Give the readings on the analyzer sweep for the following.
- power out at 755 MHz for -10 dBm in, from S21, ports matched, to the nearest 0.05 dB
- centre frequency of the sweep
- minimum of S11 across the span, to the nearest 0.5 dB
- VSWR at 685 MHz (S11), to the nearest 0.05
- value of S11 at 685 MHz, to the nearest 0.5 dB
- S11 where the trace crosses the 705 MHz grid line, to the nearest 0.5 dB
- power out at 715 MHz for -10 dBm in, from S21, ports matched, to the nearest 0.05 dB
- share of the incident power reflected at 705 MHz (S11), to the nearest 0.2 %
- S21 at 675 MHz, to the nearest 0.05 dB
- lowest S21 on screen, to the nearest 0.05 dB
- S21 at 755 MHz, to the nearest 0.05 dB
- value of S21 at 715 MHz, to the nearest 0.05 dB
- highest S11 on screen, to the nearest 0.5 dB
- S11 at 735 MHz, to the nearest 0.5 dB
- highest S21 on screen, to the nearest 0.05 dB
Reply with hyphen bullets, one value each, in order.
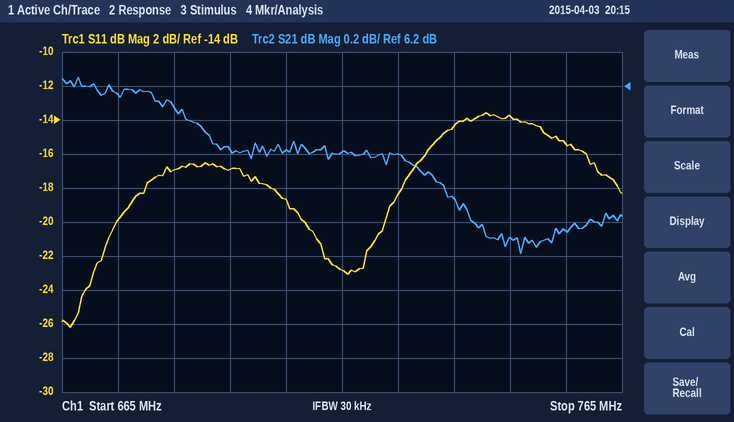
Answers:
- -4.65 dBm
- 715 MHz
- -26.0 dB
- 1.35
- -17.0 dB
- -18.5 dB
- -4.20 dBm
- 1.4 %
- 6.15 dB
- 5.20 dB
- 5.35 dB
- 5.80 dB
- -13.5 dB
- -14.5 dB
- 6.25 dB
